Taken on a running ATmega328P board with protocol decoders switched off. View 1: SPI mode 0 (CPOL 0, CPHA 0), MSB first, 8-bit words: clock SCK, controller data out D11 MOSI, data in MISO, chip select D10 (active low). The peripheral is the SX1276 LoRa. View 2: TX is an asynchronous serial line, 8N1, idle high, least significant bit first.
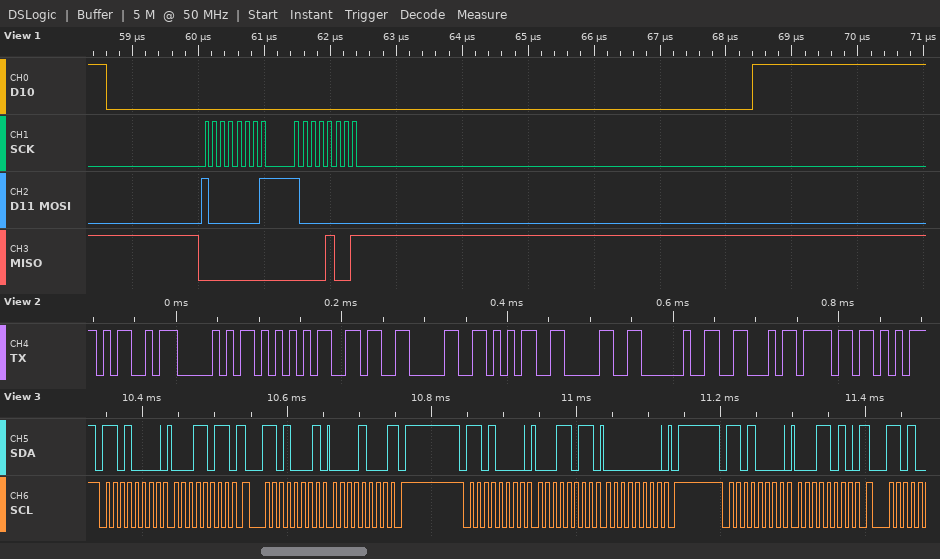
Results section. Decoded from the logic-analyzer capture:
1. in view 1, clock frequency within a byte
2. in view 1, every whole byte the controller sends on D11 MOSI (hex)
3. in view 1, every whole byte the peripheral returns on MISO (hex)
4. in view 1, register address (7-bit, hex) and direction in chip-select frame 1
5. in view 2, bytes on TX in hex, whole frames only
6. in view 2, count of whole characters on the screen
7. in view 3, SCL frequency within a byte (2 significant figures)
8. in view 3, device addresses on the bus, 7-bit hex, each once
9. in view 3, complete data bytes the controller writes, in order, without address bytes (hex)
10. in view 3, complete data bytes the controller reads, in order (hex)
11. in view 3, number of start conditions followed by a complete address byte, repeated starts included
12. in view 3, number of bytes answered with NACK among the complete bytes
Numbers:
8 MHz
0x81 0x80
0x00 0x09
0x01 write
0x4D 0x50 0x55 0x36 0x30 0x35 0x30 0x20 0x46 0x6F
10
100 kHz
0x68
1B 1B 00 1A
08
4
1
